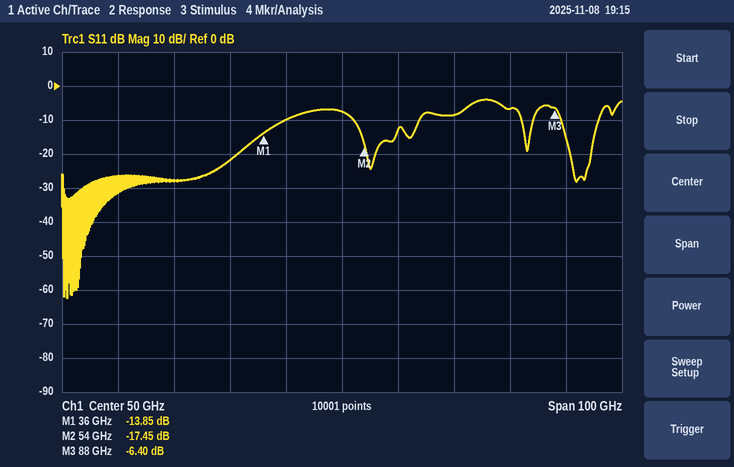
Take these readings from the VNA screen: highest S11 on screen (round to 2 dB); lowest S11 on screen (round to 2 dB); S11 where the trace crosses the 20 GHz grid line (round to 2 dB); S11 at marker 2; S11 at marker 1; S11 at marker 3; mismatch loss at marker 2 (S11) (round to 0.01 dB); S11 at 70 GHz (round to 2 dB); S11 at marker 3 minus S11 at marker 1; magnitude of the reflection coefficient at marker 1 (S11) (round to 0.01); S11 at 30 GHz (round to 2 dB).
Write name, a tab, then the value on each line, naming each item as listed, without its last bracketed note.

highest S11 on screen	-4 dB
lowest S11 on screen	-62 dB
S11 where the trace crosses the 20 GHz grid line	-28 dB
S11 at marker 2	-17.45 dB
S11 at marker 1	-13.85 dB
S11 at marker 3	-6.40 dB
mismatch loss at marker 2 (S11)	0.08 dB
S11 at 70 GHz	-8 dB
S11 at marker 3 minus S11 at marker 1	7.45 dB
magnitude of the reflection coefficient at marker 1 (S11)	0.20
S11 at 30 GHz	-22 dB
